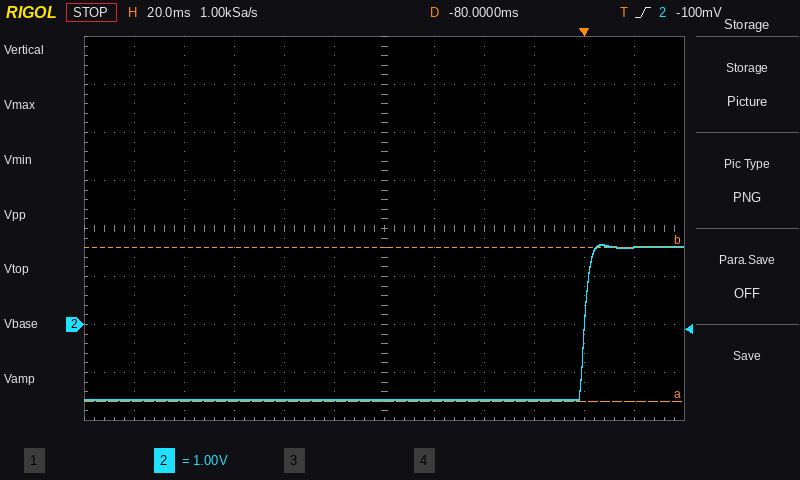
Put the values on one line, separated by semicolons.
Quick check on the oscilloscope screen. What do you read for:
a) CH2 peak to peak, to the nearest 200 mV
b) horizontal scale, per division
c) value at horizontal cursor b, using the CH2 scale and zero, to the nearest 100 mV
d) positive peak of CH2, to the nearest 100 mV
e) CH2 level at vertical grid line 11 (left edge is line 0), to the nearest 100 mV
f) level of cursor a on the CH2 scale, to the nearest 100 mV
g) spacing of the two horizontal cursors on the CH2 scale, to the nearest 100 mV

3.2 V; 20 ms; 1.6 V; 1.7 V; 1.6 V; -1.6 V; 3.2 V
